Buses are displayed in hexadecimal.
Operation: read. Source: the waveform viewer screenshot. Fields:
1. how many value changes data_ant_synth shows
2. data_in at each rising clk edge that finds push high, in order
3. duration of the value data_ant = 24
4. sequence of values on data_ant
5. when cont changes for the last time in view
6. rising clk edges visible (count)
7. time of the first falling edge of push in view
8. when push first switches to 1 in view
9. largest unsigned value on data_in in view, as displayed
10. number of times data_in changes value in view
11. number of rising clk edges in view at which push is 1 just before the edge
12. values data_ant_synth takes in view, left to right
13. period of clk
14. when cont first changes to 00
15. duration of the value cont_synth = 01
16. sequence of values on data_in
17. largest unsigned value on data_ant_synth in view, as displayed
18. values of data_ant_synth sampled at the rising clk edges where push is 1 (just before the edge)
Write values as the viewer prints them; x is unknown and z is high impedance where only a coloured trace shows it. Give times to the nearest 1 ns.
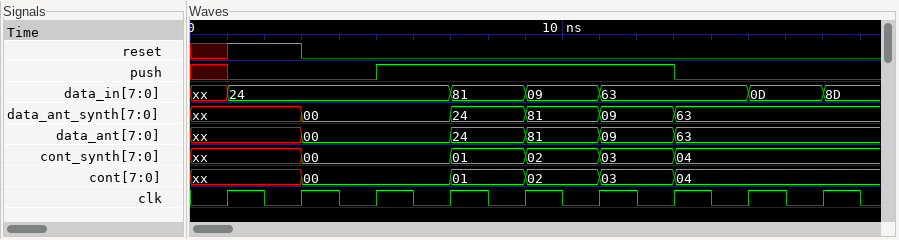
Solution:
5
24, 81, 09, 63
2 ns
xx, 00, 24, 81, 09, 63
13 ns
9
13 ns
5 ns
8D
6
4
xx, 00, 24, 81, 09, 63
2 ns
3 ns
2 ns
xx, 24, 81, 09, 63, 0D, 8D
81
00, 24, 81, 09
